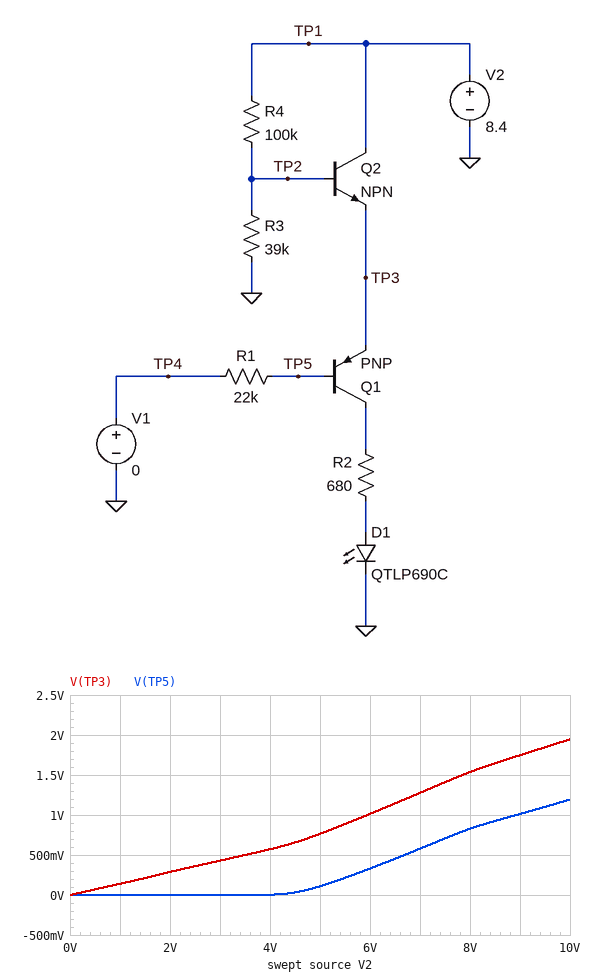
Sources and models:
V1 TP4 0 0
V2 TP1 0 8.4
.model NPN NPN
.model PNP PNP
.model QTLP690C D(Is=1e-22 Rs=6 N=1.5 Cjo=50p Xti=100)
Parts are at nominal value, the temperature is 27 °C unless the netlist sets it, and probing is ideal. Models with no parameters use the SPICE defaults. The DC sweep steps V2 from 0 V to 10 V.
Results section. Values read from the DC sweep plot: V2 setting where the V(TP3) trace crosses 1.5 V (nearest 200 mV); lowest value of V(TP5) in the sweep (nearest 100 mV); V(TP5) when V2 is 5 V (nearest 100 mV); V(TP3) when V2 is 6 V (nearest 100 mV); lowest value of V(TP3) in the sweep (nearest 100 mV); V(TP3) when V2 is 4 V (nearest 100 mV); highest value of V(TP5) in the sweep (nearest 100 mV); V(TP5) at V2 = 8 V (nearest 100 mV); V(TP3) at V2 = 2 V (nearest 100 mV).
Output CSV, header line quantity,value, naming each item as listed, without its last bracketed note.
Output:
quantity,value
V2 setting where the V(TP3) trace crosses 1.5 V,7.8 V
lowest value of V(TP5) in the sweep,0 V
V(TP5) when V2 is 5 V,100 mV
V(TP3) when V2 is 6 V,1.0 V
lowest value of V(TP3) in the sweep,0 V
V(TP3) when V2 is 4 V,600 mV
highest value of V(TP5) in the sweep,1.2 V
V(TP5) at V2 = 8 V,800 mV
V(TP3) at V2 = 2 V,300 mV
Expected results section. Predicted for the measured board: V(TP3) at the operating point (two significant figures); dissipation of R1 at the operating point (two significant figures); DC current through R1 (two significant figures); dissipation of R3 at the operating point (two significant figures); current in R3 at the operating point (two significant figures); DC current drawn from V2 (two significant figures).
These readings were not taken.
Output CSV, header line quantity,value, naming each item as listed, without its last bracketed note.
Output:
quantity,value
V(TP3) at the operating point,1.6 V
dissipation of R1 at the operating point,37 µW
DC current through R1,41 µA
dissipation of R3 at the operating point,140 µW
current in R3 at the operating point,60 µA
DC current drawn from V2,140 µA
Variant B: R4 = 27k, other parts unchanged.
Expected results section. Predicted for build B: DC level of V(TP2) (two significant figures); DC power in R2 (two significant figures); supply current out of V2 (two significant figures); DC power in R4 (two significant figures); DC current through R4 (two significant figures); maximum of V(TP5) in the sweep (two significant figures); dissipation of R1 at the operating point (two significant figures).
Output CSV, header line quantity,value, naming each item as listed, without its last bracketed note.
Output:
quantity,value
DC level of V(TP2),4.5 V
DC power in R2,5.1 mW
supply current out of V2,3.0 mA
DC power in R4,560 µW
DC current through R4,140 µA
maximum of V(TP5) in the sweep,3.7 V
dissipation of R1 at the operating point,380 µW
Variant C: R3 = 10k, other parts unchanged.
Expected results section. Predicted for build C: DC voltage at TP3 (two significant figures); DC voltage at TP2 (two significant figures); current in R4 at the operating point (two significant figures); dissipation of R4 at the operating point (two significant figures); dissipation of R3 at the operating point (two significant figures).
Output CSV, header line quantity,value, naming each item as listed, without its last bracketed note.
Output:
quantity,value
DC voltage at TP3,390 mV
DC voltage at TP2,760 mV
current in R4 at the operating point,76 µA
dissipation of R4 at the operating point,580 µW
dissipation of R3 at the operating point,58 µW
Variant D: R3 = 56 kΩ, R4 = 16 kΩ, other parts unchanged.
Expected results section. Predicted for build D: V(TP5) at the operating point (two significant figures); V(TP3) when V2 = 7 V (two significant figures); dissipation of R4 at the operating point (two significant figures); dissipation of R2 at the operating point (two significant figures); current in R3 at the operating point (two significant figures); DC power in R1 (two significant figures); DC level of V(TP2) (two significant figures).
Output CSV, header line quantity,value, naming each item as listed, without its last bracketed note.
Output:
quantity,value
V(TP5) at the operating point,4.3 V
V(TP3) when V2 = 7 V,4.2 V
dissipation of R4 at the operating point,380 µW
dissipation of R2 at the operating point,15 mW
current in R3 at the operating point,110 µA
DC power in R1,840 µW
DC level of V(TP2),5.9 V
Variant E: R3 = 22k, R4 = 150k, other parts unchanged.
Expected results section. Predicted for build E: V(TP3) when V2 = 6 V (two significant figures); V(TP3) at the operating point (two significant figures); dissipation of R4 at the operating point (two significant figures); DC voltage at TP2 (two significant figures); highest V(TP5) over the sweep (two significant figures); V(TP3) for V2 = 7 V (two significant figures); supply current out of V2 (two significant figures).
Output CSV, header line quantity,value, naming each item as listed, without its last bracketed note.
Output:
quantity,value
V(TP3) when V2 = 6 V,390 mV
V(TP3) at the operating point,550 mV
dissipation of R4 at the operating point,360 µW
DC voltage at TP2,1.1 V
highest V(TP5) over the sweep,40 mV
V(TP3) for V2 = 7 V,460 mV
supply current out of V2,49 µA
